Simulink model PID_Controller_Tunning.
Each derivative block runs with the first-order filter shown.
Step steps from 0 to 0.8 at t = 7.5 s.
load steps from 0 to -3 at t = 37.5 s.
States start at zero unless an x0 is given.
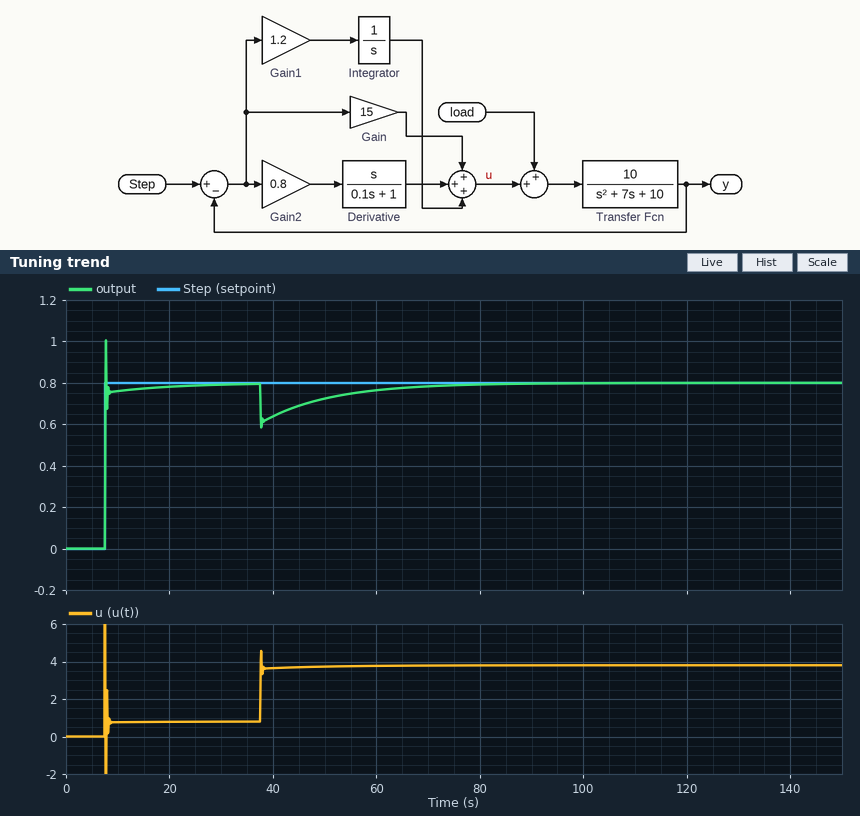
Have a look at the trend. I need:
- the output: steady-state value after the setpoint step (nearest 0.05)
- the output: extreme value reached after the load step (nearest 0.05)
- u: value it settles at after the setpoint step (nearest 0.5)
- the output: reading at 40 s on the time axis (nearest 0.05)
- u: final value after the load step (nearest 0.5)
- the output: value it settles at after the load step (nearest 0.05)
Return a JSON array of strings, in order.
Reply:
["0.80", "0.60", "1.0", "0.65", "4.0", "0.80"]
